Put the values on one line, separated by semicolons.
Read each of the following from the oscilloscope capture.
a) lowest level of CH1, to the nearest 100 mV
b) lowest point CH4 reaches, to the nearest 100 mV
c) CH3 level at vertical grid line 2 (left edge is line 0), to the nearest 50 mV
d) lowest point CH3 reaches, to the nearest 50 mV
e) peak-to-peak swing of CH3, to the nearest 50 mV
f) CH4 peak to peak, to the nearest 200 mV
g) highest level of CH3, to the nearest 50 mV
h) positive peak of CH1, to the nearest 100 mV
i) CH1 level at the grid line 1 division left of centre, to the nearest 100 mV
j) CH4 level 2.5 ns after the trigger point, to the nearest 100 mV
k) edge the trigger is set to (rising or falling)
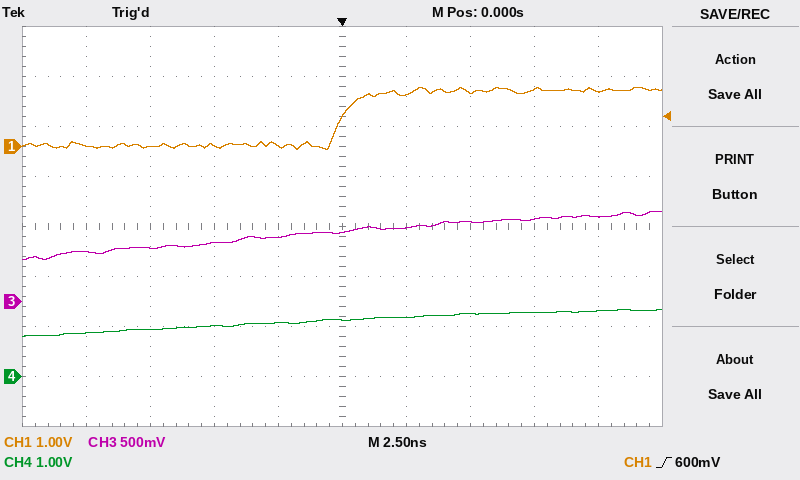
-100 mV; 800 mV; 550 mV; 400 mV; 500 mV; 600 mV; 900 mV; 1.2 V; 0.0 V; 1.2 V; rising
